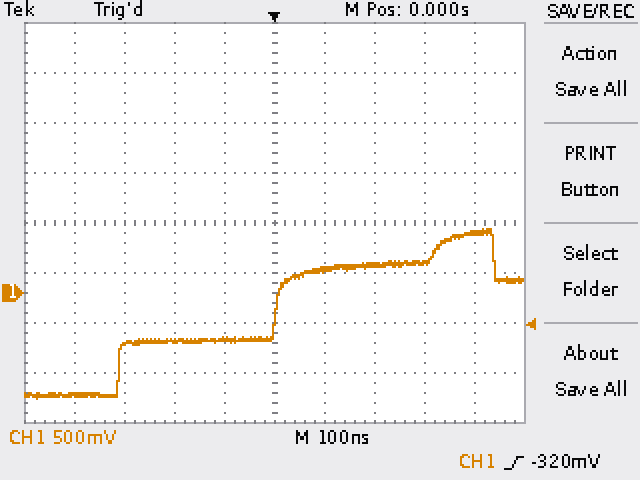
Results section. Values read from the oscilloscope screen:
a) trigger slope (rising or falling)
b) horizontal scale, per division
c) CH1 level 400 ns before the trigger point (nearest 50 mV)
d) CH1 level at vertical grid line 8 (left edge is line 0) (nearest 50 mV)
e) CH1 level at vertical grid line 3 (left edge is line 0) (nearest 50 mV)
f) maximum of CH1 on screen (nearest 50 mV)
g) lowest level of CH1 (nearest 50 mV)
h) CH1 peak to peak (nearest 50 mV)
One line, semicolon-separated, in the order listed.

rising; 100 ns; -1.00 V; 300 mV; -500 mV; 650 mV; -1.05 V; 1.70 V
